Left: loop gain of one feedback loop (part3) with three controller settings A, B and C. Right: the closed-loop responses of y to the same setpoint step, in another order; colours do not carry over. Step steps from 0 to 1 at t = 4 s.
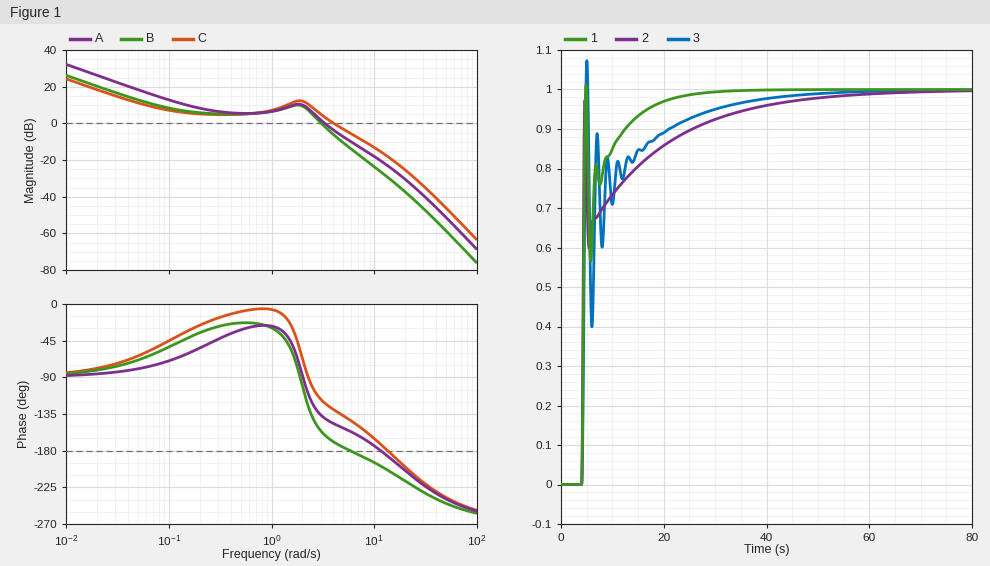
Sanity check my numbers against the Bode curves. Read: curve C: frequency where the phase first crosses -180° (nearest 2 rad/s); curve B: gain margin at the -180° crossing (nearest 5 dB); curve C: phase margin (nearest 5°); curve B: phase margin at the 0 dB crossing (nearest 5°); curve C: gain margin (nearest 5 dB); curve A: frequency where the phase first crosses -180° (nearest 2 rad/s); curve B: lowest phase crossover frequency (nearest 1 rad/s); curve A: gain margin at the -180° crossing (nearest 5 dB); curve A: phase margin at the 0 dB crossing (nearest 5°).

14 rad/s
15 dB
50°
25°
20 dB
12 rad/s
6 rad/s
20 dB
40°
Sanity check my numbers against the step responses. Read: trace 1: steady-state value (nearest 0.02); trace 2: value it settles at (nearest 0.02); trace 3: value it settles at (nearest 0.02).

1.00
1.00
1.00
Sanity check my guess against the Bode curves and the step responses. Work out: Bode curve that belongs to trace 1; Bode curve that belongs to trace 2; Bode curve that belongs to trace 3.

A
C
B
